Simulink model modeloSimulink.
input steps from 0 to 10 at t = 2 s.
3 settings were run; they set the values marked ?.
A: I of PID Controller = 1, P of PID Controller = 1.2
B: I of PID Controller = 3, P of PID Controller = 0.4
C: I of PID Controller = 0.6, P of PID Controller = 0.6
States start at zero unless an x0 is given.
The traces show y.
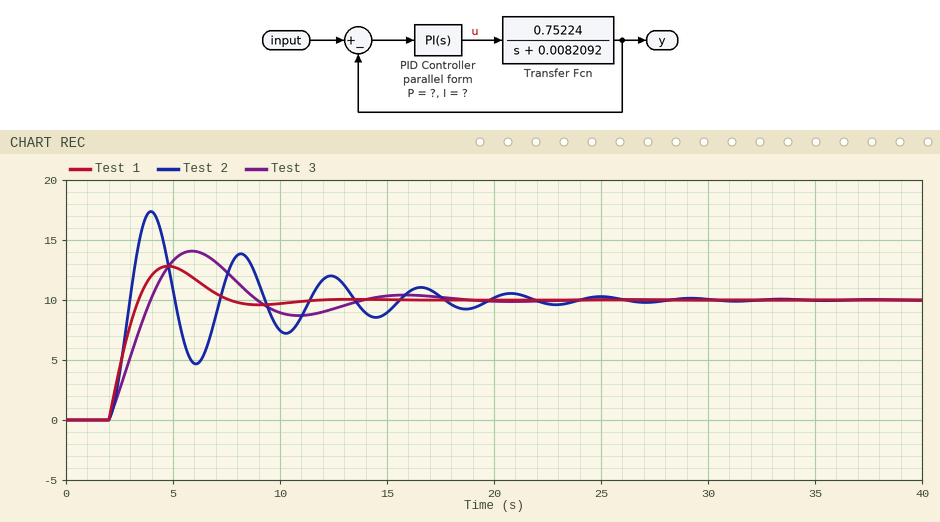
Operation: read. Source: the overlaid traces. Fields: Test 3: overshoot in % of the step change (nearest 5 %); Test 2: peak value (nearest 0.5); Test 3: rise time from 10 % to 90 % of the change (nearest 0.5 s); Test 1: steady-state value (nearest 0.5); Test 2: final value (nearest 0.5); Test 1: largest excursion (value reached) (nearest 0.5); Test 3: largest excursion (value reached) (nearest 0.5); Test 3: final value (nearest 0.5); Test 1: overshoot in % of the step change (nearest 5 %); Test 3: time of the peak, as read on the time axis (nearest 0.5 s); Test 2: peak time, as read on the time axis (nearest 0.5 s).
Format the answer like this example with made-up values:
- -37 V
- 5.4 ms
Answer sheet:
- 40 %
- 17.5
- 1.5 s
- 10.0
- 10.0
- 13.0
- 14.0
- 10.0
- 30 %
- 6.0 s
- 4.0 s
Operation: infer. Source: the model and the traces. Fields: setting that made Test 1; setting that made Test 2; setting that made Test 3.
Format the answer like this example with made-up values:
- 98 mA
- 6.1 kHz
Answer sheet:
- A
- B
- C
